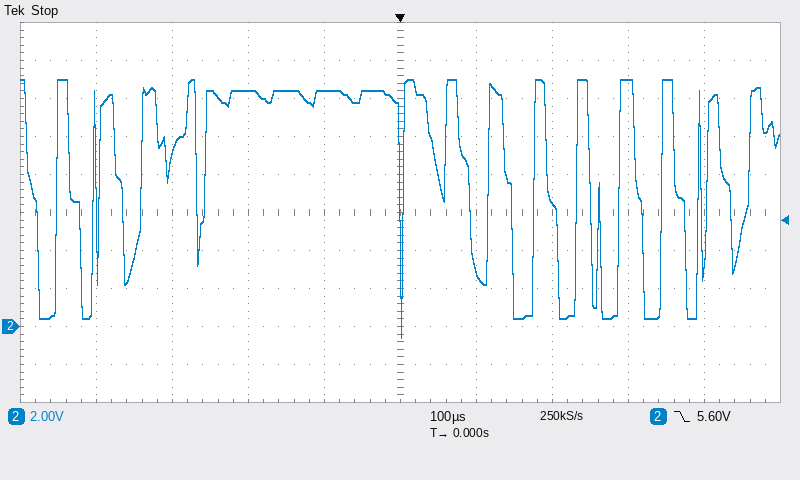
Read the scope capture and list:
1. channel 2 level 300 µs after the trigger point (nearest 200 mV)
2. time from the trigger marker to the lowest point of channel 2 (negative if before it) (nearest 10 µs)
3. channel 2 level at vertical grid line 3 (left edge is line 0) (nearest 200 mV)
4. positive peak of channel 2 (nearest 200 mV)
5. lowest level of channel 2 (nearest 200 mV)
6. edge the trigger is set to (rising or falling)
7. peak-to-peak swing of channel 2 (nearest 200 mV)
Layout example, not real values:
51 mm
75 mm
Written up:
13.0 V
0 µs
12.4 V
13.0 V
-600 mV
falling
13.6 V
